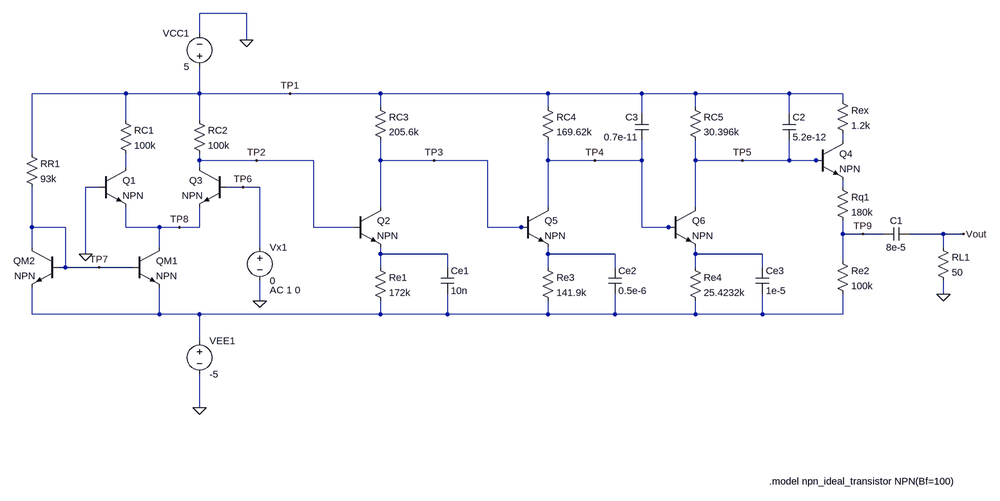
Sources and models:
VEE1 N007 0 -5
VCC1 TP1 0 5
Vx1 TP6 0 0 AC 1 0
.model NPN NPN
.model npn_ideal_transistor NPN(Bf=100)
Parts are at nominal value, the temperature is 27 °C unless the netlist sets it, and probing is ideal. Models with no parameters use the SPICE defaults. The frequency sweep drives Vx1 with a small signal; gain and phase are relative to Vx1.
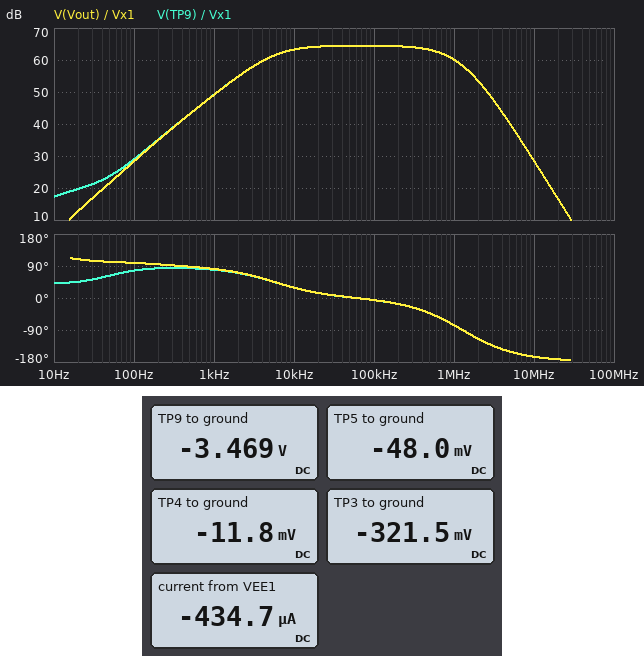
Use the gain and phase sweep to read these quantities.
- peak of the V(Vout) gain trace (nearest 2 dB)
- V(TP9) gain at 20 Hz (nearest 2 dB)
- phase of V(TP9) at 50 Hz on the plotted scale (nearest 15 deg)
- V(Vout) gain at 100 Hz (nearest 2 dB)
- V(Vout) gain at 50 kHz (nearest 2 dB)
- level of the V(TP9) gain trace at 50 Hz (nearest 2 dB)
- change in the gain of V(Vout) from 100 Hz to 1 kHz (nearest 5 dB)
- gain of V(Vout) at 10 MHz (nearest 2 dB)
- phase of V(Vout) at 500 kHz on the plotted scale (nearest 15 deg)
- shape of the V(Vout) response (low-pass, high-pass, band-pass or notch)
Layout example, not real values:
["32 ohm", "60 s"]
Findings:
["64 dB", "20 dB", "60 deg", "28 dB", "64 dB", "24 dB", "20 dB", "28 dB", "-45 deg", "band-pass"]
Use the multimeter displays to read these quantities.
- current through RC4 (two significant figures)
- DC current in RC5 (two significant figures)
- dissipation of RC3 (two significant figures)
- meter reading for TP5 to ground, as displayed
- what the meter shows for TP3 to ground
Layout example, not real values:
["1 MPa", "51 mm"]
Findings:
["30 µA", "170 µA", "140 µW", "-48.0 mV", "-321.5 mV"]
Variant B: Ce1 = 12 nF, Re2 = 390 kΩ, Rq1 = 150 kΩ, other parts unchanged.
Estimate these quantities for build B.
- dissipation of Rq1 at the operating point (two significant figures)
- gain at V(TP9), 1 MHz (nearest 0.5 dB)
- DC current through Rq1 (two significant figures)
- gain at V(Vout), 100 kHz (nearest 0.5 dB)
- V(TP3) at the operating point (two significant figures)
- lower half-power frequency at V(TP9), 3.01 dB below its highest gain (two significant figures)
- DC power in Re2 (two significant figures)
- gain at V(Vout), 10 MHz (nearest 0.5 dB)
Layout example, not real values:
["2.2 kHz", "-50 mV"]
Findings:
["9.5 µW", "61.5 dB", "8.0 µA", "66.0 dB", "-320 mV", "4.8 kHz", "25 µW", "30.0 dB"]
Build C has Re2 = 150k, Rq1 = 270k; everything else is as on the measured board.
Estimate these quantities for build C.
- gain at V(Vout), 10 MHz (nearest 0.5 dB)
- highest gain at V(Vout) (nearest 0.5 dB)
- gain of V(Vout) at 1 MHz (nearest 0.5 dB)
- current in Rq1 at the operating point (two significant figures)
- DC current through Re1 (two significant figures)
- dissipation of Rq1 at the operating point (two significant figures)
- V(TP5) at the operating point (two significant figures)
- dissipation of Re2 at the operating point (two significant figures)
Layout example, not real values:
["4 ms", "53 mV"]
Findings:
["25.0 dB", "61.0 dB", "56.5 dB", "10 µA", "26 µA", "28 µW", "-46 mV", "16 µW"]
